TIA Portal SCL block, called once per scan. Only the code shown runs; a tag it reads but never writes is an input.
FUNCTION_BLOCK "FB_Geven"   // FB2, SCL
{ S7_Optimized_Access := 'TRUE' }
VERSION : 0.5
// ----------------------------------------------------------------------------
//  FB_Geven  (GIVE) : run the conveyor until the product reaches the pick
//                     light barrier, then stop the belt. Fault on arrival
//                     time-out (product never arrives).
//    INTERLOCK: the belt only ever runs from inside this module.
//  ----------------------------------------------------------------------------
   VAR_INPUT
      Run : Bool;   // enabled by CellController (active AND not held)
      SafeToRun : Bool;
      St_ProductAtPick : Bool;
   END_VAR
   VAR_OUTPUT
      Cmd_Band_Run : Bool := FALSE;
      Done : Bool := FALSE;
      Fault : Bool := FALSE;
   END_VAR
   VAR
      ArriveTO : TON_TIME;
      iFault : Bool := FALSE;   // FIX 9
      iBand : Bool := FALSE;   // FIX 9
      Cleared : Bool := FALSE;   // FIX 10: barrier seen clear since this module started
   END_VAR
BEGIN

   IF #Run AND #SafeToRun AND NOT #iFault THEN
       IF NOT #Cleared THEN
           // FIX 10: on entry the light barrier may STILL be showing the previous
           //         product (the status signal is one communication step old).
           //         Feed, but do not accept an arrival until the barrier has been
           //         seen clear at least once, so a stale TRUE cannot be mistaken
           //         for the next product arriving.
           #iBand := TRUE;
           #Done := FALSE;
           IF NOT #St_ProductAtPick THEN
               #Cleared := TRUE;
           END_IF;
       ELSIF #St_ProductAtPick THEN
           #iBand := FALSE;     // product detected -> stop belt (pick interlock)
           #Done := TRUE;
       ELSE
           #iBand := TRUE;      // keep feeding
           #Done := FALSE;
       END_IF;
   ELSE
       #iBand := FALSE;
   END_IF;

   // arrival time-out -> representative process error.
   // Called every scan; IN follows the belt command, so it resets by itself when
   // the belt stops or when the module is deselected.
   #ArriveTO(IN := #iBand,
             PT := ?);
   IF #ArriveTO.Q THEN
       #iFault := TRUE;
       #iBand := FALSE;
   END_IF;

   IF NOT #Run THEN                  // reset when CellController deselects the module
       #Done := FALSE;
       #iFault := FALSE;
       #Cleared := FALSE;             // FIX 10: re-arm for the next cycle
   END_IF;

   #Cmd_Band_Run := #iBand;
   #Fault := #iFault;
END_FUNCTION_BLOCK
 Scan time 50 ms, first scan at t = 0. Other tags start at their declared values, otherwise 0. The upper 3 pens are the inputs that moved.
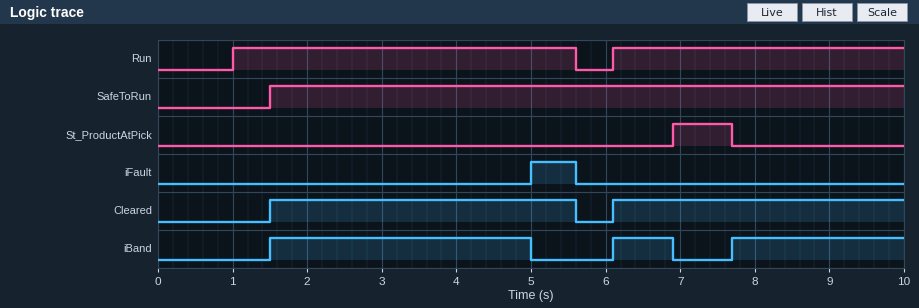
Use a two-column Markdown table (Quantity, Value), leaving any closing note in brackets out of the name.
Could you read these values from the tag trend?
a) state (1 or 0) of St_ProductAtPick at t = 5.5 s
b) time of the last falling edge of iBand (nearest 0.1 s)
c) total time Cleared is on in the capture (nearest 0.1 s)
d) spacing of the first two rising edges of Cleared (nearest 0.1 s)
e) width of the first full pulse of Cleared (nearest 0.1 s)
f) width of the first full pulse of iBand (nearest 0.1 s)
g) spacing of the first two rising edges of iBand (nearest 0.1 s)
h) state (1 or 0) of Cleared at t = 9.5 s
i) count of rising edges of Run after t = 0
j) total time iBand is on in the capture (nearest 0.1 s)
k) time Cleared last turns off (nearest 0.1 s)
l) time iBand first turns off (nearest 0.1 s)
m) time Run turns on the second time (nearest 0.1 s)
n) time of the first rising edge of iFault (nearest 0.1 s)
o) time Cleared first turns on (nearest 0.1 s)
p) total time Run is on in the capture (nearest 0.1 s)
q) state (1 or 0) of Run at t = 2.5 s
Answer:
| Quantity | Value |
|---|---|
| state (1 or 0) of St_ProductAtPick at t = 5.5 s | 0 |
| time of the last falling edge of iBand | 6.9 s |
| total time Cleared is on in the capture | 8.0 s |
| spacing of the first two rising edges of Cleared | 4.6 s |
| width of the first full pulse of Cleared | 4.1 s |
| width of the first full pulse of iBand | 3.5 s |
| spacing of the first two rising edges of iBand | 4.6 s |
| state (1 or 0) of Cleared at t = 9.5 s | 1 |
| count of rising edges of Run after t = 0 | 2 |
| total time iBand is on in the capture | 6.6 s |
| time Cleared last turns off | 5.6 s |
| time iBand first turns off | 5.0 s |
| time Run turns on the second time | 6.1 s |
| time of the first rising edge of iFault | 5.0 s |
| time Cleared first turns on | 1.5 s |
| total time Run is on in the capture | 8.5 s |
| state (1 or 0) of Run at t = 2.5 s | 1 |
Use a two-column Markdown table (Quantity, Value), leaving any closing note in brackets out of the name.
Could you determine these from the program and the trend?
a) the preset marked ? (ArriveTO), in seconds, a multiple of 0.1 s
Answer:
| Quantity | Value |
|---|---|
| the preset marked ? (ArriveTO), in seconds, a multiple of 0.1 s | 3.5 s |
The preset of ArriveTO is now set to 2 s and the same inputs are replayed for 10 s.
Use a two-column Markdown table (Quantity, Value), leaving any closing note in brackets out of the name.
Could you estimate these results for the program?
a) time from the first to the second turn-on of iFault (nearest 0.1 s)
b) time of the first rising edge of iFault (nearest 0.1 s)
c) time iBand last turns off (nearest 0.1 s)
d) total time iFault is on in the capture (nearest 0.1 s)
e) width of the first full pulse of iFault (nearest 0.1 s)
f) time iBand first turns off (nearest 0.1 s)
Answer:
| Quantity | Value |
|---|---|
| time from the first to the second turn-on of iFault | 6.2 s |
| time of the first rising edge of iFault | 3.5 s |
| time iBand last turns off | 9.7 s |
| total time iFault is on in the capture | 2.4 s |
| width of the first full pulse of iFault | 2.1 s |
| time iBand first turns off | 3.5 s |
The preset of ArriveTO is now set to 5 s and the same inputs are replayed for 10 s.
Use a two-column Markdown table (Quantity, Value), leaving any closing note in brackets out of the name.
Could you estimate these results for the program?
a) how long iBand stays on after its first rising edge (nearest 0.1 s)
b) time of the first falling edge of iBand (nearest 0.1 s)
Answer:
| Quantity | Value |
|---|---|
| how long iBand stays on after its first rising edge | 4.1 s |
| time of the first falling edge of iBand | 5.6 s |
